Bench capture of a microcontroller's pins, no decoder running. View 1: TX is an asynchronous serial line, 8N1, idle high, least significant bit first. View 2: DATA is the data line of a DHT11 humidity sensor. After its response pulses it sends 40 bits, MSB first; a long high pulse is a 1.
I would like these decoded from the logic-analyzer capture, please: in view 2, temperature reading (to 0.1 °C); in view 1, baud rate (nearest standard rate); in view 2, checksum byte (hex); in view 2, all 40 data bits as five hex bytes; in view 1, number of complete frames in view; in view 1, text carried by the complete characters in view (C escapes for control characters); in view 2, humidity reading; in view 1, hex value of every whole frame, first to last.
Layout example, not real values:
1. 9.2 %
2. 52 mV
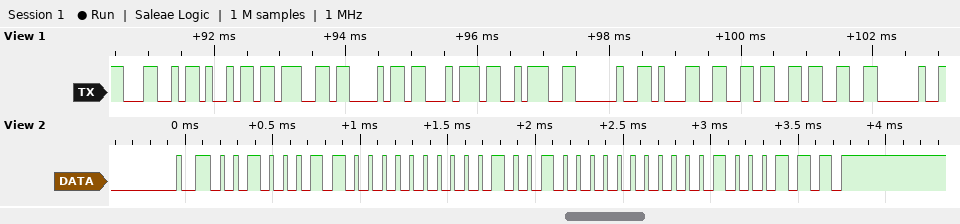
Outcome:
1. 36.0 °C
2. 9600 baud
3. 0x47
4. 23 00 24 00 47
5. 11
6. "Light: 163 "
7. 35 %
8. 4C 69 67 68 74 3A 20 31 36 33 20
